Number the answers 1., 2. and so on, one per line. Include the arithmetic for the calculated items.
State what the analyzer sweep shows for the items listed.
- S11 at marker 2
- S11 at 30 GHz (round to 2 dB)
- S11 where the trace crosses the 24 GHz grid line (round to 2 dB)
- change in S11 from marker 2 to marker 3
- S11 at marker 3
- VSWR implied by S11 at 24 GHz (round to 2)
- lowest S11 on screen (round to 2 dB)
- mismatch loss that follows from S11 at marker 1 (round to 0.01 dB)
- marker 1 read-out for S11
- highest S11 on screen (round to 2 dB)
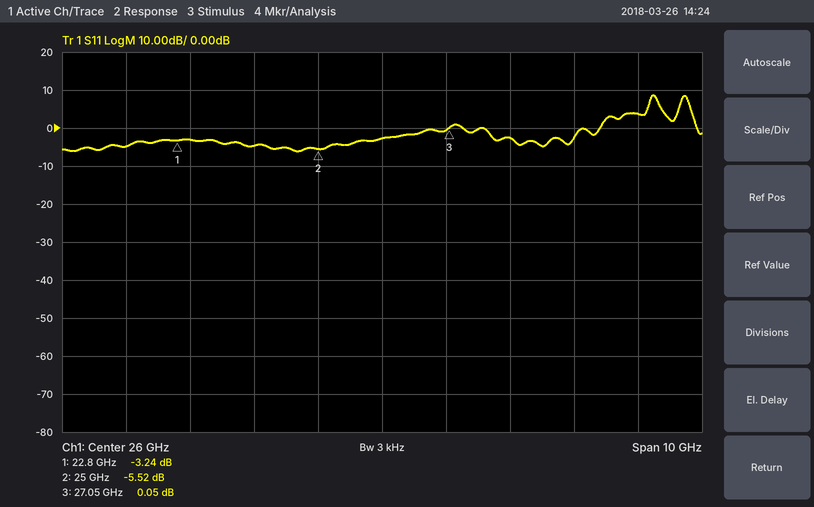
1. -5.52 dB
2. 4 dB
3. -4 dB
4. 0.05 − (-5.52) = 5.57 dB
5. 0.05 dB
6. |Γ| = 10^(-4/20) = 0.6310; VSWR = (1 + 0.6310)/(1 − 0.6310) ≈ 4
7. -6 dB
8. −10 log10(1 − 10^(-3.24/10)) ≈ 2.79 dB
9. -3.24 dB
10. 8 dB
